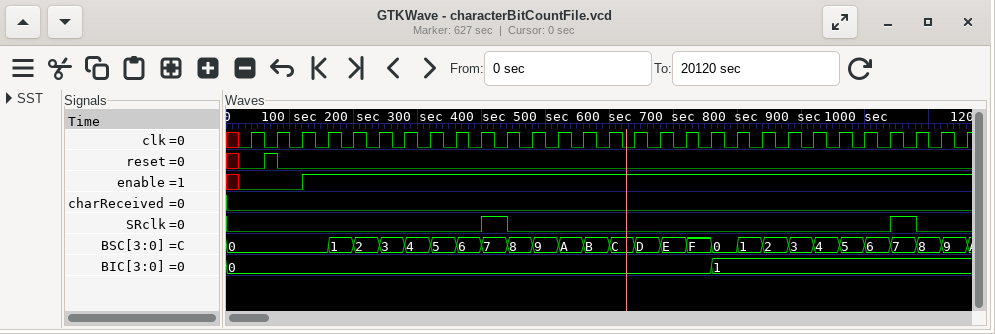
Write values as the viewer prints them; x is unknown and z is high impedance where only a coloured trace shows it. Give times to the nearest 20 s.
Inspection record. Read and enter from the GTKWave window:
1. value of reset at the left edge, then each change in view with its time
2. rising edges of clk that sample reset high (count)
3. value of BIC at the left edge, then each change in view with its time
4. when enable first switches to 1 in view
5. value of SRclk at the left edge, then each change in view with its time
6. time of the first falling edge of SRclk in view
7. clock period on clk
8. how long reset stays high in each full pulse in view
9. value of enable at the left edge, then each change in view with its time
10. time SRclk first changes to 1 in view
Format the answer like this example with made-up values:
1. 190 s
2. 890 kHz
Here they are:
1. x, 0 at 20 s, 1 at 60 s, 0 at 80 s
2. 1
3. 0, 1 at 760 s
4. 120 s
5. 0, 1 at 400 s, 0 at 440 s, 1 at 1040 s, 0 at 1080 s
6. 440 s
7. 40 s
8. 20 s
9. x, 0 at 20 s, 1 at 120 s
10. 400 s
